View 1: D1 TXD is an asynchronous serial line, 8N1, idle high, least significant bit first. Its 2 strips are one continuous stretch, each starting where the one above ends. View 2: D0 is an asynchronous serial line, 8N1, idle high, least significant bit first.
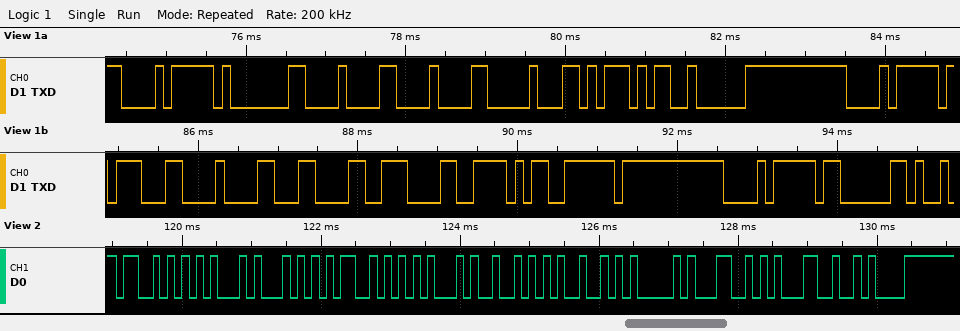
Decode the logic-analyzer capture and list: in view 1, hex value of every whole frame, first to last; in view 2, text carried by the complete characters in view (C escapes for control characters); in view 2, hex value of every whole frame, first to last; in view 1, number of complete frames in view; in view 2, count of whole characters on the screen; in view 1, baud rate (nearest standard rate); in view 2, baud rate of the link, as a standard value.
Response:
0xE8 0x01 0x08 0x08 0x10 0x5D 0x02 0xE8 0x1D 0x08 0x0C 0x0E 0x5E 0x7E 0xE8 0x03
"SETSERIAL1\n"
0x53 0x45 0x54 0x53 0x45 0x52 0x49 0x41 0x4C 0x31 0x0A
16
11
9600 baud
9600 baud
